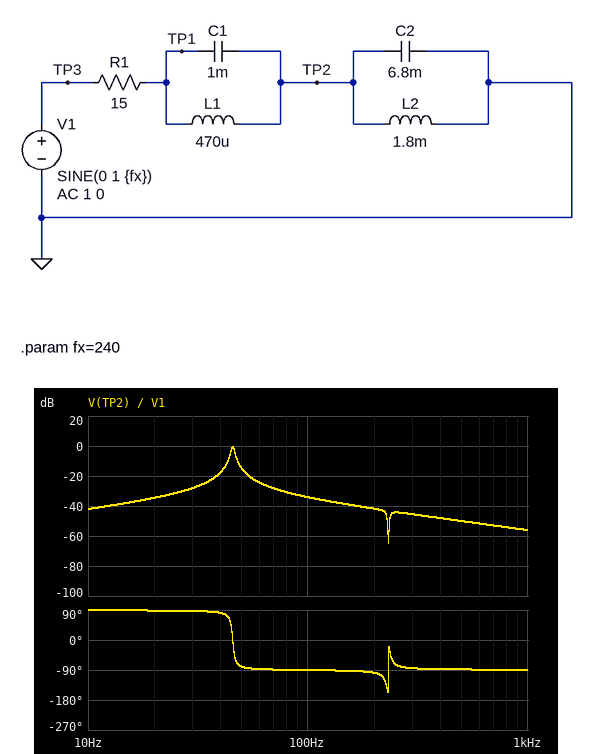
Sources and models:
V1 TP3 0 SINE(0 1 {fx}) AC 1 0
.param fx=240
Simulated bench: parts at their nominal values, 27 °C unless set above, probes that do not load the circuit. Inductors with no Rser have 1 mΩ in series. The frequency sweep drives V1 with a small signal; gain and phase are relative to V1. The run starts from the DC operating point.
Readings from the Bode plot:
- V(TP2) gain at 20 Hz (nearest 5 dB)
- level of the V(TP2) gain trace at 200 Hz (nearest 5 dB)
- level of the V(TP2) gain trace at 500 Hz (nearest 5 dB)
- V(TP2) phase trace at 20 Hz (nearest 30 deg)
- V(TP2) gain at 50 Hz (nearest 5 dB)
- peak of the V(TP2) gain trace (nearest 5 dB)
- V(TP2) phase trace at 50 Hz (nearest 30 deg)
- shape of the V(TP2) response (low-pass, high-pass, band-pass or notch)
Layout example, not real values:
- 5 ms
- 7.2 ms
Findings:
- -35 dB
- -40 dB
- -50 dB
- 90 deg
- -15 dB
- 0 dB
- -90 deg
- band-pass
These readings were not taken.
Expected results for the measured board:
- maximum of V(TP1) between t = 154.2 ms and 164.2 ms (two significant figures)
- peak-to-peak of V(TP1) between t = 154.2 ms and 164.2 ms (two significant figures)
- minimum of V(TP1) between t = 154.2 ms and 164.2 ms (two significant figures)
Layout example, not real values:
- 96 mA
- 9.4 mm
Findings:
- 570 mV
- 1.1 V
- -570 mV
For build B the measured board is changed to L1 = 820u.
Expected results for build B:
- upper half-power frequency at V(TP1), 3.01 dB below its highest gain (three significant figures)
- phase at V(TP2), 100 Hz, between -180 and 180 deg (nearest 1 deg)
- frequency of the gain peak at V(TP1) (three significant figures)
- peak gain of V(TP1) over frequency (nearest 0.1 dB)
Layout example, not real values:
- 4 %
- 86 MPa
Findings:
- 181 Hz
- -92 deg
- 176 Hz
- -0.2 dB
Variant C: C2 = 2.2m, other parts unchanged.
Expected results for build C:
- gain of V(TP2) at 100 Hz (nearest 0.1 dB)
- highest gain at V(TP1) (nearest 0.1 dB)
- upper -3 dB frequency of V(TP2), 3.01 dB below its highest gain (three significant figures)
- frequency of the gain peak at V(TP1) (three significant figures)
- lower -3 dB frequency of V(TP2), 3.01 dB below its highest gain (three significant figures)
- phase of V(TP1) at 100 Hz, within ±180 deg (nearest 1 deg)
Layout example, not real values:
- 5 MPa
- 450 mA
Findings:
- -17.5 dB
- -0.2 dB
- 82.5 Hz
- 80.0 Hz
- 77.6 Hz
- -84 deg
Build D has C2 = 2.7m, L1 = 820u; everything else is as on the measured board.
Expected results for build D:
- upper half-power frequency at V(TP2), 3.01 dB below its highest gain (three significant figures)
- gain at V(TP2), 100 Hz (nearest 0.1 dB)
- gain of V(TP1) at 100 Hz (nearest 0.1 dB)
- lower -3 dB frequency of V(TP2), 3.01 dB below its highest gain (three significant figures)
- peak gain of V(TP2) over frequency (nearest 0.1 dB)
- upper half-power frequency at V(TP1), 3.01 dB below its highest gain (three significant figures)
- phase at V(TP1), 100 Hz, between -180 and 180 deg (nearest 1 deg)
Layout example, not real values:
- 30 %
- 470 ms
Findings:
- 74.3 Hz
- -21.7 dB
- -30.1 dB
- 70.3 Hz
- -0.2 dB
- 181 Hz
- -88 deg
